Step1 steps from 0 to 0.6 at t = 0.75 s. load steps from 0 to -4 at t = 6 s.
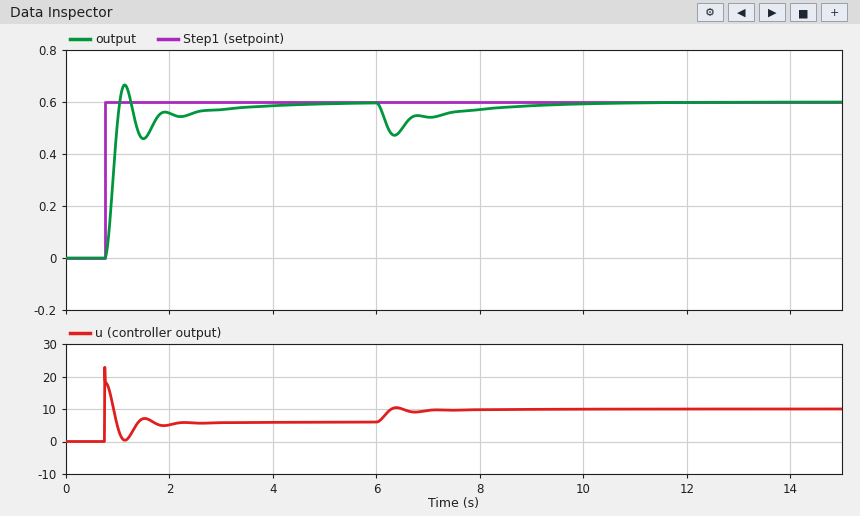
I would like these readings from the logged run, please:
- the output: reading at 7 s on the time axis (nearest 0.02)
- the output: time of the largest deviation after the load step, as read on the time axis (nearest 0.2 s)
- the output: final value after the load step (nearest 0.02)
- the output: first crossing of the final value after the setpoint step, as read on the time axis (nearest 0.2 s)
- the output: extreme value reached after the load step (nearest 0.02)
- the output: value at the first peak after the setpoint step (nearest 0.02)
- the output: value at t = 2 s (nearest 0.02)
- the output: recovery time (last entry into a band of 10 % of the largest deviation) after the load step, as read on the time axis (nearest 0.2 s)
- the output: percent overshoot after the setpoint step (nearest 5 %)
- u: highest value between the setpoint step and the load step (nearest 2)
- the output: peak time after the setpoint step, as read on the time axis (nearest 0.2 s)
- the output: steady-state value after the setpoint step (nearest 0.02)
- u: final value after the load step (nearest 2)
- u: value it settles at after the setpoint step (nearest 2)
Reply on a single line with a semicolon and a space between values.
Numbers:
0.54; 6.4 s; 0.60; 1.0 s; 0.48; 0.66; 0.56; 9.2 s; 10 %; 22; 1.2 s; 0.60; 10; 6
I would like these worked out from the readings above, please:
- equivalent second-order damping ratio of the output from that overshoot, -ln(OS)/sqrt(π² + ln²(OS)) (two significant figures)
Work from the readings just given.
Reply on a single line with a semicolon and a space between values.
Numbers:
0.59
